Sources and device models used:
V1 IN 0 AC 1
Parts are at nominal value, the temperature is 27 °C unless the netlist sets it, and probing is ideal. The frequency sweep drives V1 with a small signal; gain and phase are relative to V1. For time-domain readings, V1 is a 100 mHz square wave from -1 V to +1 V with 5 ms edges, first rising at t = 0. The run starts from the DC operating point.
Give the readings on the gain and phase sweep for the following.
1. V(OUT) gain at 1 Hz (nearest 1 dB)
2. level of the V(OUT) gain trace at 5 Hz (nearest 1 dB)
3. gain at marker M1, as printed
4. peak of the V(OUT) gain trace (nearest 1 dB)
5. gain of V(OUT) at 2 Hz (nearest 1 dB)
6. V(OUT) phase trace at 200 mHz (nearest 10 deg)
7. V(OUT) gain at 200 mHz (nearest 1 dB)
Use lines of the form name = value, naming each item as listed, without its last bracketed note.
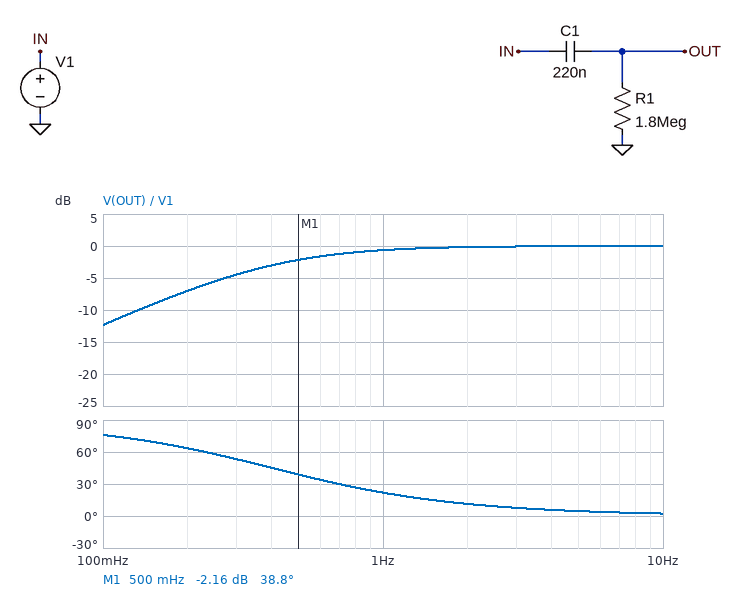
V(OUT) gain at 1 Hz = -1 dB
level of the V(OUT) gain trace at 5 Hz = 0 dB
gain at marker M1, as printed = -2.16 dB
peak of the V(OUT) gain trace = 0 dB
gain of V(OUT) at 2 Hz = 0 dB
V(OUT) phase trace at 200 mHz = 60 deg
V(OUT) gain at 200 mHz = -7 dB
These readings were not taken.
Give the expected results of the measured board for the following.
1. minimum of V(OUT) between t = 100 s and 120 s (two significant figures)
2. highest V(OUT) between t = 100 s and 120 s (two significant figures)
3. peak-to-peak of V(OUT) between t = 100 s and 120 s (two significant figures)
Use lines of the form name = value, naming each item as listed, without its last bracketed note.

minimum of V(OUT) between t = 100 s and 120 s = -2.0 V
highest V(OUT) between t = 100 s and 120 s = 2.0 V
peak-to-peak of V(OUT) between t = 100 s and 120 s = 4.0 V
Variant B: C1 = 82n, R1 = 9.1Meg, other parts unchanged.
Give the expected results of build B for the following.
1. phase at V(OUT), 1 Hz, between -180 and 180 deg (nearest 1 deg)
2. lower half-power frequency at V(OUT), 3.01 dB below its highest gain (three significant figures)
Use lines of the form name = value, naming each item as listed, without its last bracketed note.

phase at V(OUT), 1 Hz, between -180 and 180 deg = 12 deg
lower half-power frequency at V(OUT), 3.01 dB below its highest gain = 213 mHz
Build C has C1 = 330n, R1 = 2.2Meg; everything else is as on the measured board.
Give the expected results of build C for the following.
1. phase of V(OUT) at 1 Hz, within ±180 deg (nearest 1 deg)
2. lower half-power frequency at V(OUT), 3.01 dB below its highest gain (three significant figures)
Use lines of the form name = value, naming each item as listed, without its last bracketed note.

phase of V(OUT) at 1 Hz, within ±180 deg = 12 deg
lower half-power frequency at V(OUT), 3.01 dB below its highest gain = 219 mHz
